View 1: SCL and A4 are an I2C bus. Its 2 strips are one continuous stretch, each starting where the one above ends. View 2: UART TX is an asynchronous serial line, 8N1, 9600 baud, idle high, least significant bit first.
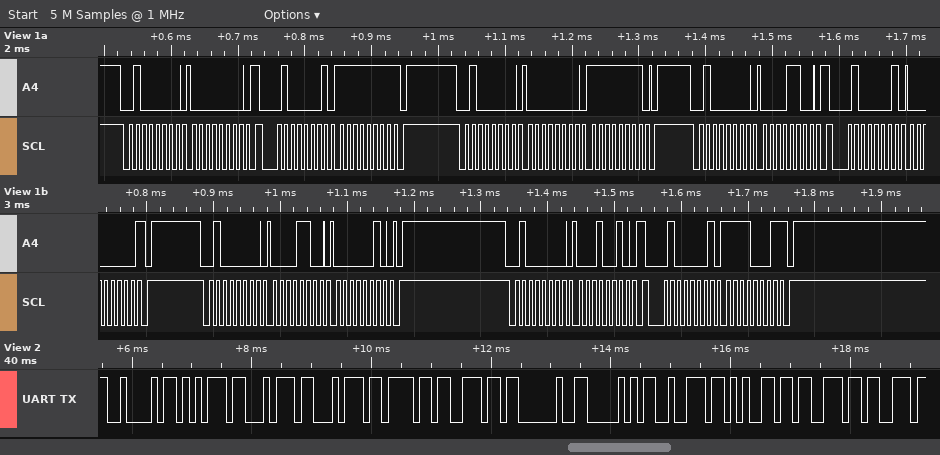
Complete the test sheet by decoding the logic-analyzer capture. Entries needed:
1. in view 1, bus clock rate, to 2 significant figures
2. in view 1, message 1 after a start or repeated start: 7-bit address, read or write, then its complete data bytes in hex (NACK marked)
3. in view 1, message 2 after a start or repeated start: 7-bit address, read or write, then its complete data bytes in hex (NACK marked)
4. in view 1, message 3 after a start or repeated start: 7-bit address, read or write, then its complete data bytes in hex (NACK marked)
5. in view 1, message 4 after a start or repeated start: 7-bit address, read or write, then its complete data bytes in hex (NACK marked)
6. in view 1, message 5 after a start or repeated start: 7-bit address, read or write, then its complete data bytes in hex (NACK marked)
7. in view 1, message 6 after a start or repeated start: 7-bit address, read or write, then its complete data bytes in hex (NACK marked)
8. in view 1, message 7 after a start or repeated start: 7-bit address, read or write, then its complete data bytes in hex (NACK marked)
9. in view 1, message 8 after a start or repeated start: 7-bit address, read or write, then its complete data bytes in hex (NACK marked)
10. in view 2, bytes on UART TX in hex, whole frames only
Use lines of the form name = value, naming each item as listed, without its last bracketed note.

in view 1, bus clock rate, to 2 significant figures = 100 kHz
in view 1, message 1 after a start or repeated start: 7-bit address, read or write, then its complete data bytes in hex = 0x20 write: 00
in view 1, message 2 after a start or repeated start: 7-bit address, read or write, then its complete data bytes in hex = 0x20 read: FF NACK
in view 1, message 3 after a start or repeated start: 7-bit address, read or write, then its complete data bytes in hex = 0x20 write: 00 FF
in view 1, message 4 after a start or repeated start: 7-bit address, read or write, then its complete data bytes in hex = 0x20 write: 0C
in view 1, message 5 after a start or repeated start: 7-bit address, read or write, then its complete data bytes in hex = 0x20 read: 00 NACK
in view 1, message 6 after a start or repeated start: 7-bit address, read or write, then its complete data bytes in hex = 0x20 write: 0C 02
in view 1, message 7 after a start or repeated start: 7-bit address, read or write, then its complete data bytes in hex = 0x20 write: 12
in view 1, message 8 after a start or repeated start: 7-bit address, read or write, then its complete data bytes in hex = 0x20 read: F1 NACK
in view 2, bytes on UART TX in hex, whole frames only = 42 75 74 74 6F 6E 20 50 72 65 73 73
